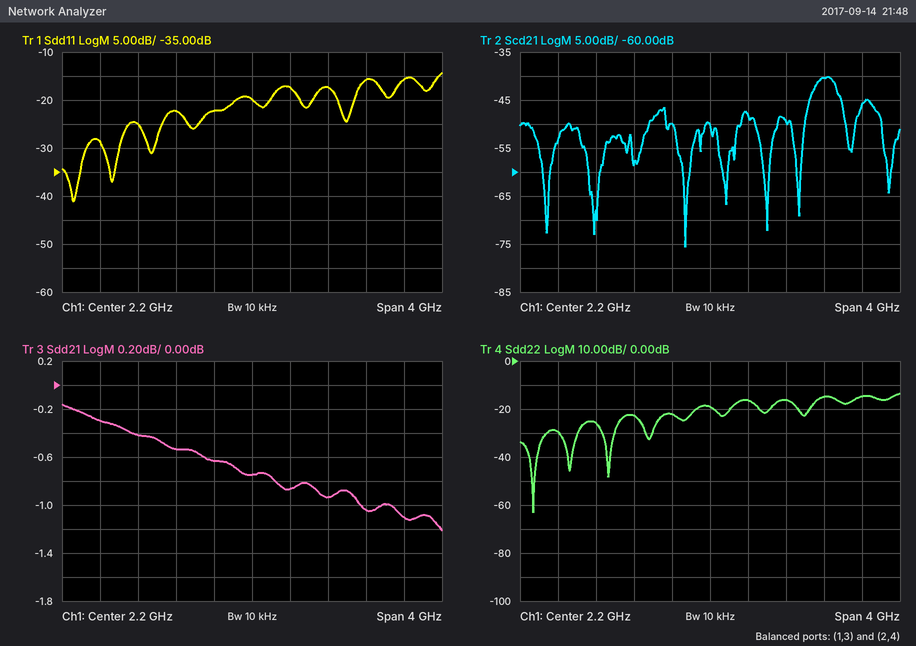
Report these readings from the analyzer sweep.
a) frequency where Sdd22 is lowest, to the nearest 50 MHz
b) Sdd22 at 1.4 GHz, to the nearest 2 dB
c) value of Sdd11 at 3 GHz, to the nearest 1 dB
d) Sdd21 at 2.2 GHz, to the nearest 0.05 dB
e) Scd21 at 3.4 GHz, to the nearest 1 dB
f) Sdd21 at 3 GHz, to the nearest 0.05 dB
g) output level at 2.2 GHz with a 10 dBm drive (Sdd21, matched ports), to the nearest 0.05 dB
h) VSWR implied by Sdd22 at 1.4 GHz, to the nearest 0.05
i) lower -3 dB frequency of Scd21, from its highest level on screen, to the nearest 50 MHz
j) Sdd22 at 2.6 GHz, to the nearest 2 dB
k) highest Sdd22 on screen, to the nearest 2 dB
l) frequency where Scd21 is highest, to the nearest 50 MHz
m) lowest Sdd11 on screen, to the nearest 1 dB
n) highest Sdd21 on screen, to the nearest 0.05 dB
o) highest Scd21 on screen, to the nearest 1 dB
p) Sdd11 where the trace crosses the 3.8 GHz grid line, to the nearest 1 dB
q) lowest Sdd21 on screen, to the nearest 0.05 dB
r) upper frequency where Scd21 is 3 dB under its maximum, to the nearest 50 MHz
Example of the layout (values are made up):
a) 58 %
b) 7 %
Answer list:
a) 350 MHz
b) -22 dB
c) -17 dB
d) -0.75 dB
e) -40 dB
f) -0.95 dB
g) 9.25 dBm
h) 1.15
i) 3.30 GHz
j) -16 dB
k) -14 dB
l) 3.45 GHz
m) -41 dB
n) -0.15 dB
o) -40 dB
p) -16 dB
q) -1.20 dB
r) 3.55 GHz
